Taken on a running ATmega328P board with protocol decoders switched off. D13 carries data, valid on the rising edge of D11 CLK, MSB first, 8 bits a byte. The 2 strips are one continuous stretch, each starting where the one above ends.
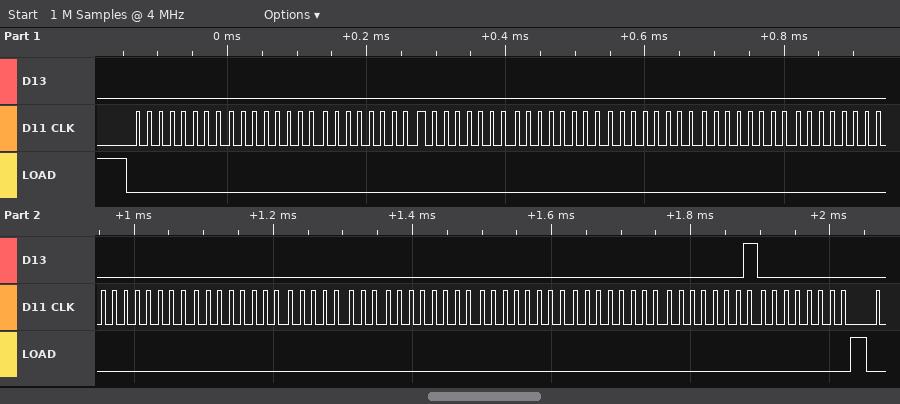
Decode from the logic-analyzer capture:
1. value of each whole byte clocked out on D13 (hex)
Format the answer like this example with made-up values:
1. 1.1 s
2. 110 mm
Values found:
1. 0x00 0x00 0x00 0x00 0x00 0x00 0x00 0x00 0x00 0x00 0x00 0x00 0x00 0x00 0x01 0x00
